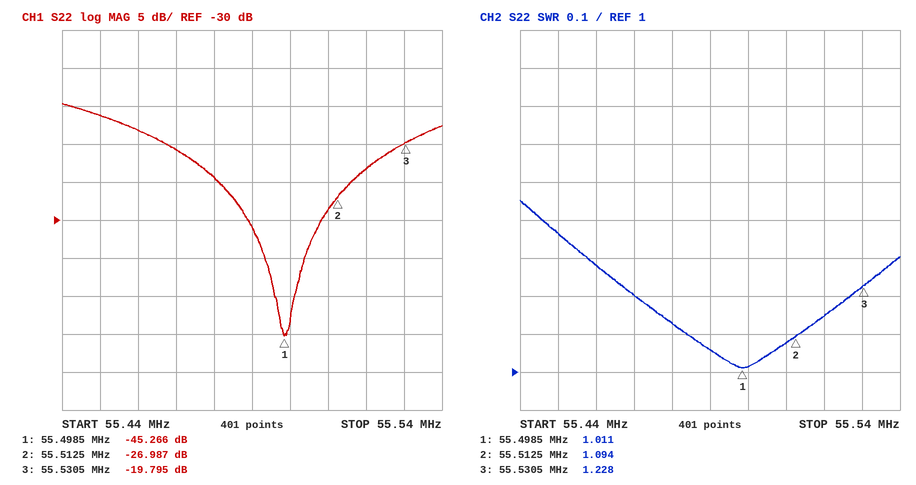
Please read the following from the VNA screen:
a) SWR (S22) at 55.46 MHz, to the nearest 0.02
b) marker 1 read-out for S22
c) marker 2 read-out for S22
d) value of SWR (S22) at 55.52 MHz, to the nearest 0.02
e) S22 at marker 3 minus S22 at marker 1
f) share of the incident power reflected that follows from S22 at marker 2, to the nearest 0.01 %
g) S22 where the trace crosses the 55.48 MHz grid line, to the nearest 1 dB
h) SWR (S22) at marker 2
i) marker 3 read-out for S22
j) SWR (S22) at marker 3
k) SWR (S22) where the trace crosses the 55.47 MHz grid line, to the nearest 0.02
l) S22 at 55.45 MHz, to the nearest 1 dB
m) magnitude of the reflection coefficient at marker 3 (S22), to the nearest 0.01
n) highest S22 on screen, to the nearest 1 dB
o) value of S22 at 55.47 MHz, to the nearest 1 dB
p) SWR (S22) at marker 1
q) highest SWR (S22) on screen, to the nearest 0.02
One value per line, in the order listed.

1.28
-45.266 dB
-26.987 dB
1.14
25.471 dB
0.20 %
-24 dB
1.094
-19.795 dB
1.228
1.20
-16 dB
0.10
-15 dB
-21 dB
1.011
1.46
